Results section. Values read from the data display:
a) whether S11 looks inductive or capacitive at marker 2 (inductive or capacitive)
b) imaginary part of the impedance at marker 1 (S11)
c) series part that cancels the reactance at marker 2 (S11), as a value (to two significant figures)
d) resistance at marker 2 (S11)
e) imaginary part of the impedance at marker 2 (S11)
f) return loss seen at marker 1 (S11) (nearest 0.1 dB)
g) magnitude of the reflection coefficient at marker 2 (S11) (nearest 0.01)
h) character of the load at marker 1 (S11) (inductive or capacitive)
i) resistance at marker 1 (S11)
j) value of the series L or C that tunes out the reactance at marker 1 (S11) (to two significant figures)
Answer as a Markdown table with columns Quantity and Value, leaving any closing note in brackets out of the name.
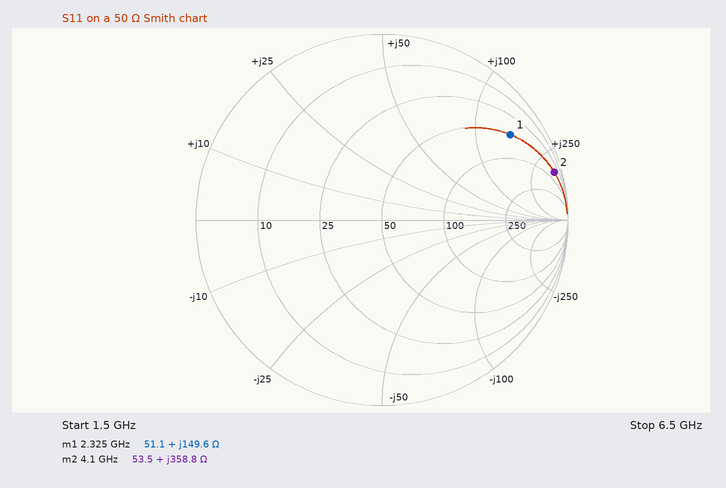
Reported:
| Quantity | Value |
|---|---|
| whether S11 looks inductive or capacitive at marker 2 | inductive |
| imaginary part of the impedance at marker 1 | +149.6 Ω |
| series part that cancels the reactance at marker 2 (S11), as a value | 110 fF |
| resistance at marker 2 | 53.5 Ω |
| imaginary part of the impedance at marker 2 | +358.8 Ω |
| return loss seen at marker 1 (S11) | 1.6 dB |
| magnitude of the reflection coefficient at marker 2 (S11) | 0.96 |
| character of the load at marker 1 (S11) | inductive |
| resistance at marker 1 | 51.1 Ω |
| value of the series L or C that tunes out the reactance at marker 1 (S11) | 460 fF |
